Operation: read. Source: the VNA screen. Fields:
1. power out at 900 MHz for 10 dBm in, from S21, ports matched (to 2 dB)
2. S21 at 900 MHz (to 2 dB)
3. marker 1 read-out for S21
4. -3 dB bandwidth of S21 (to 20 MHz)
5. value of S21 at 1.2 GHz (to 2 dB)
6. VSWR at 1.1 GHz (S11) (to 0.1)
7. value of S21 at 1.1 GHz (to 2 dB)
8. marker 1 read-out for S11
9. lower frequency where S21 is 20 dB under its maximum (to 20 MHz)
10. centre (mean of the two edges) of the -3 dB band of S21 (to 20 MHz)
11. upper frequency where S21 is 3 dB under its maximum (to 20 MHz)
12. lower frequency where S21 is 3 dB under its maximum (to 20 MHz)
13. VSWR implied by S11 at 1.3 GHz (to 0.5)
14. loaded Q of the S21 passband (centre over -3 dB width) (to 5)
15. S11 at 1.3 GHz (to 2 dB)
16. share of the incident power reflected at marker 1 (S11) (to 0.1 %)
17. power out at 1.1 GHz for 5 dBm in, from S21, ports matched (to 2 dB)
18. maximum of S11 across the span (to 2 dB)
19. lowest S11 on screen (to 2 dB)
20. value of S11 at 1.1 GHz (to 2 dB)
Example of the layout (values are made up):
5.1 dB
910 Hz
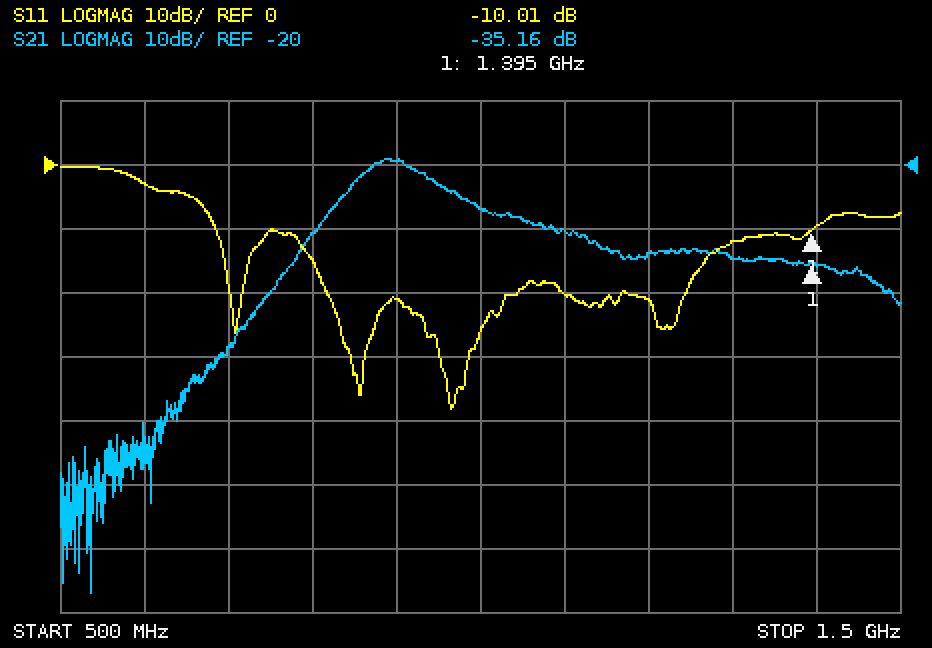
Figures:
-10 dBm
-20 dB
-35.16 dB
80 MHz
-34 dB
1.2
-30 dB
-10.01 dB
760 MHz
900 MHz
940 MHz
860 MHz
1.5
10
-12 dB
10.0 %
-26 dBm
0 dB
-38 dB
-20 dB
